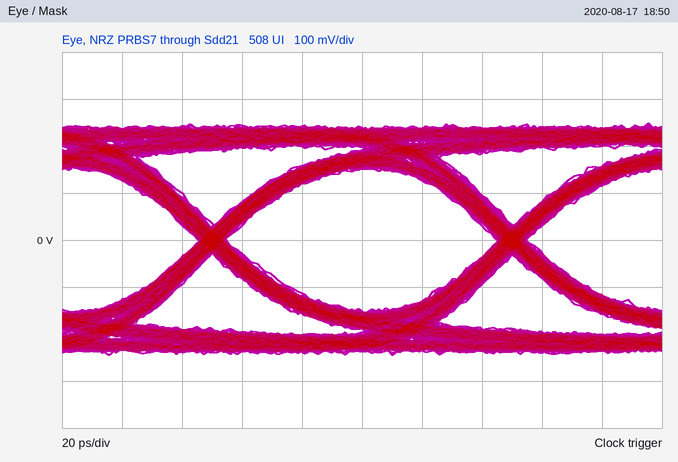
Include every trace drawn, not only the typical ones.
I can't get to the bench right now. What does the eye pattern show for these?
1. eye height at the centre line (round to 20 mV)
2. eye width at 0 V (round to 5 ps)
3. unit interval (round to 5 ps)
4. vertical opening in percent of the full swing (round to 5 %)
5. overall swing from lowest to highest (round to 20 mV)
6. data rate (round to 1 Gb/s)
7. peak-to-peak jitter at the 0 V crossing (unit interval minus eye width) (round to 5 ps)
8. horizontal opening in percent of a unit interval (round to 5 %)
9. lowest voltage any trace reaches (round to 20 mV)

300 mV
90 ps
100 ps
60 %
500 mV
10 Gb/s
10 ps
90 %
-240 mV
